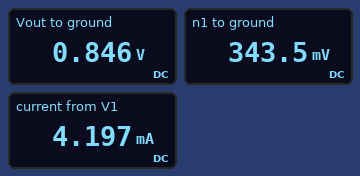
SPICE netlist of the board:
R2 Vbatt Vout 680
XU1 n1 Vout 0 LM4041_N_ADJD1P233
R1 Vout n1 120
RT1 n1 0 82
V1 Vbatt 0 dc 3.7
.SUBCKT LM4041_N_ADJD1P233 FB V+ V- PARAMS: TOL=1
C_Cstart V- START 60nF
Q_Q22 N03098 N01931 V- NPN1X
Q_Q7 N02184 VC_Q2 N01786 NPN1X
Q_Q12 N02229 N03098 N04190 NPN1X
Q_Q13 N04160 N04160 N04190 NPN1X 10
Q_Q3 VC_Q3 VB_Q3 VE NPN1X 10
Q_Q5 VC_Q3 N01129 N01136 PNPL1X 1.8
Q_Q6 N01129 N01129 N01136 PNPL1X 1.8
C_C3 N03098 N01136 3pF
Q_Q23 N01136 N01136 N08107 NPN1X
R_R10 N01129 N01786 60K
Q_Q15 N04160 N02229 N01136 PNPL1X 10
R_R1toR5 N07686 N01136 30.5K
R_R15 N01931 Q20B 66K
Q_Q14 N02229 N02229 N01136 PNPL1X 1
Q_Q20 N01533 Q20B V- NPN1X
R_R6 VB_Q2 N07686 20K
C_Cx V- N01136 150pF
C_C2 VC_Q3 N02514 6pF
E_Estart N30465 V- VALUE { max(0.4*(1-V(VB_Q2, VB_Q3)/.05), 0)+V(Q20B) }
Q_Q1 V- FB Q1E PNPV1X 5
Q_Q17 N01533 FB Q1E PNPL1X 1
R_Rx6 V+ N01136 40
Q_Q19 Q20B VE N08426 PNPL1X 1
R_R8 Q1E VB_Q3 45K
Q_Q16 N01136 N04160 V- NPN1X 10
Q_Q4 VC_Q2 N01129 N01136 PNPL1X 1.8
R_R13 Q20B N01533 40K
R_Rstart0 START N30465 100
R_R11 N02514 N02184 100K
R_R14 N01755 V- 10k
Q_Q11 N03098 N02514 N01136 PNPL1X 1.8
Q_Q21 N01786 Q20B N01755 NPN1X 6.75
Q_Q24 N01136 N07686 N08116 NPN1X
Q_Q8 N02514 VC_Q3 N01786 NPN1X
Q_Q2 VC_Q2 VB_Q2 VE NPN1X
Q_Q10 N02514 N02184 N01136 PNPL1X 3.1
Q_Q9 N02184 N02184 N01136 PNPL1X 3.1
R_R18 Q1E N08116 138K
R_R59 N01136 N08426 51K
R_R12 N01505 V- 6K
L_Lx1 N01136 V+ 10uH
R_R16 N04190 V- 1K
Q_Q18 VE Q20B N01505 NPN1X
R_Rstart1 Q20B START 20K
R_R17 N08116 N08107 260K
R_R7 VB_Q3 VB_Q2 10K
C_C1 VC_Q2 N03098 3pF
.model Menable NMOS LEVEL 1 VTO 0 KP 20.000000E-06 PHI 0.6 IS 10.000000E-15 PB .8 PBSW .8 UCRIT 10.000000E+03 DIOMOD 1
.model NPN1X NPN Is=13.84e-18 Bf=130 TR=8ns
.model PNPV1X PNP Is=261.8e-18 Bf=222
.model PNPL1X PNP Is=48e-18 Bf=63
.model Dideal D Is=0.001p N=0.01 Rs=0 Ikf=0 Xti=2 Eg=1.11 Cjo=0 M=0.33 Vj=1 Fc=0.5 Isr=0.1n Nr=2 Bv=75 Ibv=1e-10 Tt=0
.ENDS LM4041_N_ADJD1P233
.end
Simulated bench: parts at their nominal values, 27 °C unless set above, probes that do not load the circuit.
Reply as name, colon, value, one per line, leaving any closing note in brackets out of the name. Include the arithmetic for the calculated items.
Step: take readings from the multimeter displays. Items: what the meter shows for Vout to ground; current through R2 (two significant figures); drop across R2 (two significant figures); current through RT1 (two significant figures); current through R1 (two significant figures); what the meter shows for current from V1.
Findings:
what the meter shows for Vout to ground: 0.846 V
current through R2: (3.7 V - 846 mV) / 680 Ω = 4.2 mA
drop across R2: 3.7 V - 846 mV = 2.9 V
current through RT1: (343.5 mV) / 82 Ω = 4.2 mA
current through R1: (846 mV - 343.5 mV) / 120 Ω = 4.2 mA
what the meter shows for current from V1: 4.197 mA
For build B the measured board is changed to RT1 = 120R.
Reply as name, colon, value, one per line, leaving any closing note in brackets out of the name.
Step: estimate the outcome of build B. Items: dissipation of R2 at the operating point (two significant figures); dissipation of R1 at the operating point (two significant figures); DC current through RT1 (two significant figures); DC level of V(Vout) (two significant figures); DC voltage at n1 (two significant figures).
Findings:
dissipation of R2 at the operating point: 11 mW
dissipation of R1 at the operating point: 1.9 mW
DC current through RT1: 4.0 mA
DC level of V(Vout): 960 mV
DC voltage at n1: 480 mV
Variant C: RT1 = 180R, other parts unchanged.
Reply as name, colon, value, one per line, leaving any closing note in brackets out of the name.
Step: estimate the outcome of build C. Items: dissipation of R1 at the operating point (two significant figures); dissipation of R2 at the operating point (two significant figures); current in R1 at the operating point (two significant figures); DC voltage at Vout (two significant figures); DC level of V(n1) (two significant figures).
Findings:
dissipation of R1 at the operating point: 1.7 mW
dissipation of R2 at the operating point: 9.7 mW
current in R1 at the operating point: 3.8 mA
DC voltage at Vout: 1.1 V
DC level of V(n1): 680 mV
